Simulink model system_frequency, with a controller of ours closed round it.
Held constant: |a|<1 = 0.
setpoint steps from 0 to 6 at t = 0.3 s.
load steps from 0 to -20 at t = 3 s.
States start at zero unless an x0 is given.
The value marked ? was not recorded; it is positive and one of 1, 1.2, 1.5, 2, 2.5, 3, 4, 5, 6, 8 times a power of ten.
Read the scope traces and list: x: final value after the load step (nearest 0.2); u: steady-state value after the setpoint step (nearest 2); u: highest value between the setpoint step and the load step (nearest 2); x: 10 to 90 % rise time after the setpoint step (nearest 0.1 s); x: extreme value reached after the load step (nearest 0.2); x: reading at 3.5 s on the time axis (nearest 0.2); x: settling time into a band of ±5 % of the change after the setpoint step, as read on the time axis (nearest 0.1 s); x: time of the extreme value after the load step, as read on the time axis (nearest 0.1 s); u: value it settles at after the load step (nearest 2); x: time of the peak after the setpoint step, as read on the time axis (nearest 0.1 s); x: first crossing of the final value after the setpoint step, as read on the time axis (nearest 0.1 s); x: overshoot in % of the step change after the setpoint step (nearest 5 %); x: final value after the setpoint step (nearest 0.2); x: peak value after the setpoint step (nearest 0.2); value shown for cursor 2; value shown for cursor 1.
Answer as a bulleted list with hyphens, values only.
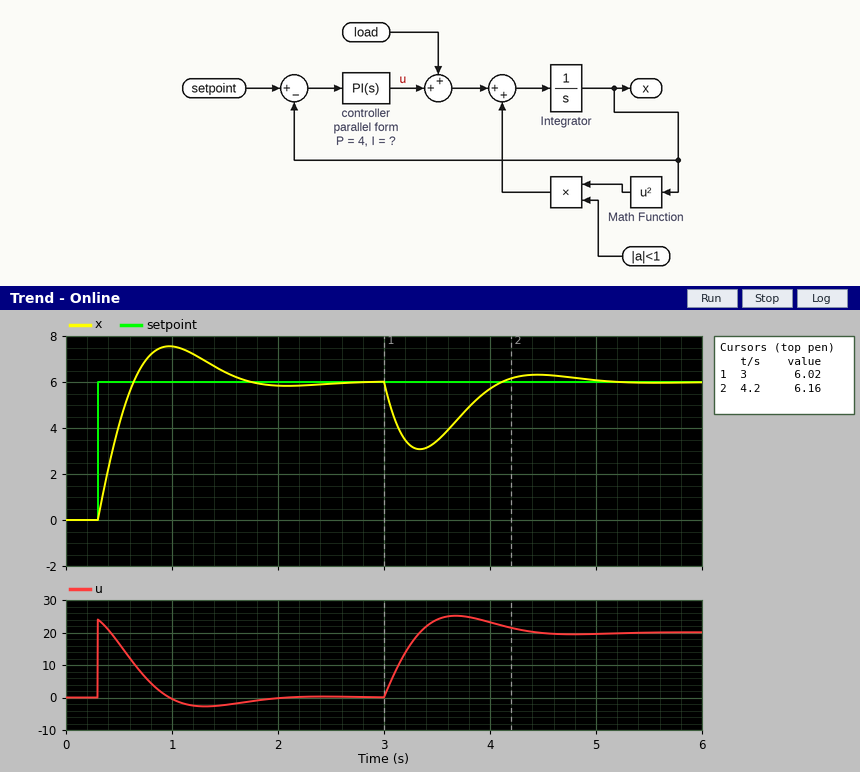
- 6.0
- 0
- 24
- 0.3 s
- 3.0
- 3.4
- 1.6 s
- 3.3 s
- 20
- 1.0 s
- 0.6 s
- 25 %
- 6.0
- 7.6
- 6.16
- 6.02
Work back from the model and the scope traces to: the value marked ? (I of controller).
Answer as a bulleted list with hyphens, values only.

- 12
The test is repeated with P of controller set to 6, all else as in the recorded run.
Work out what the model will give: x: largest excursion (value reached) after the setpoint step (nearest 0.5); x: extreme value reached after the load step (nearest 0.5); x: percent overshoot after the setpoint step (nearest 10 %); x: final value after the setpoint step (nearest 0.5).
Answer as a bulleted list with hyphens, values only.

- 7.0
- 3.5
- 20 %
- 6.0
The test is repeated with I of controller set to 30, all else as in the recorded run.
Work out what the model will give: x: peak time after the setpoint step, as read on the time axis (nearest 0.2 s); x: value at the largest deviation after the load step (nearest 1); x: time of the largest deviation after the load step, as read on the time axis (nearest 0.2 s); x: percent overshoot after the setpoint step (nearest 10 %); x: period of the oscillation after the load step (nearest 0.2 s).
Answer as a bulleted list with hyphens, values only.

- 0.8 s
- 4
- 3.2 s
- 40 %
- 1.2 s
